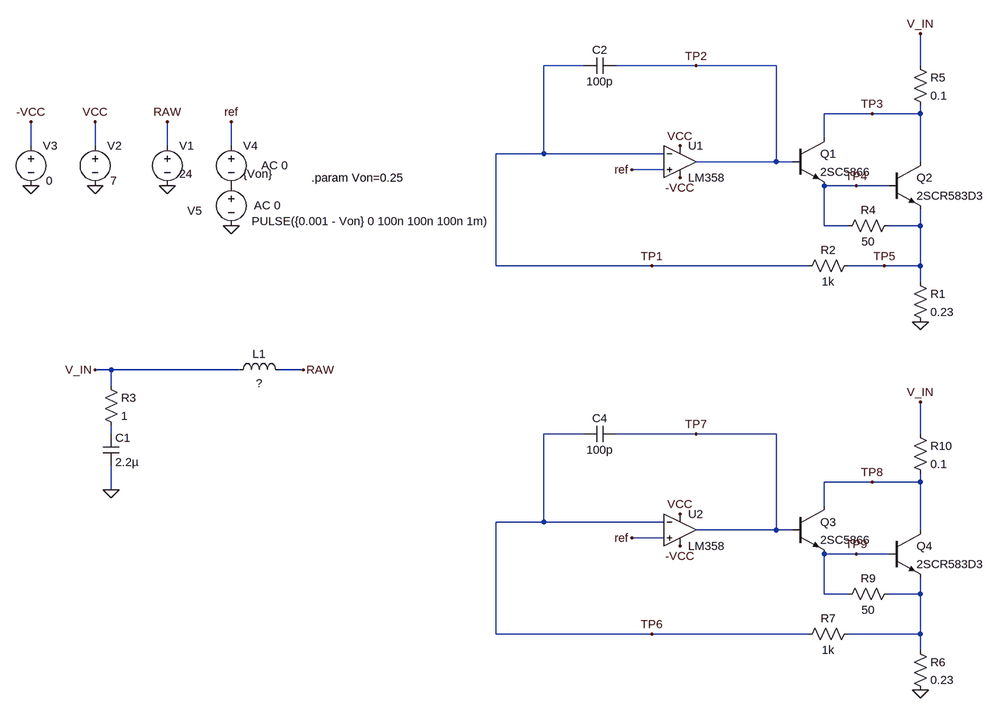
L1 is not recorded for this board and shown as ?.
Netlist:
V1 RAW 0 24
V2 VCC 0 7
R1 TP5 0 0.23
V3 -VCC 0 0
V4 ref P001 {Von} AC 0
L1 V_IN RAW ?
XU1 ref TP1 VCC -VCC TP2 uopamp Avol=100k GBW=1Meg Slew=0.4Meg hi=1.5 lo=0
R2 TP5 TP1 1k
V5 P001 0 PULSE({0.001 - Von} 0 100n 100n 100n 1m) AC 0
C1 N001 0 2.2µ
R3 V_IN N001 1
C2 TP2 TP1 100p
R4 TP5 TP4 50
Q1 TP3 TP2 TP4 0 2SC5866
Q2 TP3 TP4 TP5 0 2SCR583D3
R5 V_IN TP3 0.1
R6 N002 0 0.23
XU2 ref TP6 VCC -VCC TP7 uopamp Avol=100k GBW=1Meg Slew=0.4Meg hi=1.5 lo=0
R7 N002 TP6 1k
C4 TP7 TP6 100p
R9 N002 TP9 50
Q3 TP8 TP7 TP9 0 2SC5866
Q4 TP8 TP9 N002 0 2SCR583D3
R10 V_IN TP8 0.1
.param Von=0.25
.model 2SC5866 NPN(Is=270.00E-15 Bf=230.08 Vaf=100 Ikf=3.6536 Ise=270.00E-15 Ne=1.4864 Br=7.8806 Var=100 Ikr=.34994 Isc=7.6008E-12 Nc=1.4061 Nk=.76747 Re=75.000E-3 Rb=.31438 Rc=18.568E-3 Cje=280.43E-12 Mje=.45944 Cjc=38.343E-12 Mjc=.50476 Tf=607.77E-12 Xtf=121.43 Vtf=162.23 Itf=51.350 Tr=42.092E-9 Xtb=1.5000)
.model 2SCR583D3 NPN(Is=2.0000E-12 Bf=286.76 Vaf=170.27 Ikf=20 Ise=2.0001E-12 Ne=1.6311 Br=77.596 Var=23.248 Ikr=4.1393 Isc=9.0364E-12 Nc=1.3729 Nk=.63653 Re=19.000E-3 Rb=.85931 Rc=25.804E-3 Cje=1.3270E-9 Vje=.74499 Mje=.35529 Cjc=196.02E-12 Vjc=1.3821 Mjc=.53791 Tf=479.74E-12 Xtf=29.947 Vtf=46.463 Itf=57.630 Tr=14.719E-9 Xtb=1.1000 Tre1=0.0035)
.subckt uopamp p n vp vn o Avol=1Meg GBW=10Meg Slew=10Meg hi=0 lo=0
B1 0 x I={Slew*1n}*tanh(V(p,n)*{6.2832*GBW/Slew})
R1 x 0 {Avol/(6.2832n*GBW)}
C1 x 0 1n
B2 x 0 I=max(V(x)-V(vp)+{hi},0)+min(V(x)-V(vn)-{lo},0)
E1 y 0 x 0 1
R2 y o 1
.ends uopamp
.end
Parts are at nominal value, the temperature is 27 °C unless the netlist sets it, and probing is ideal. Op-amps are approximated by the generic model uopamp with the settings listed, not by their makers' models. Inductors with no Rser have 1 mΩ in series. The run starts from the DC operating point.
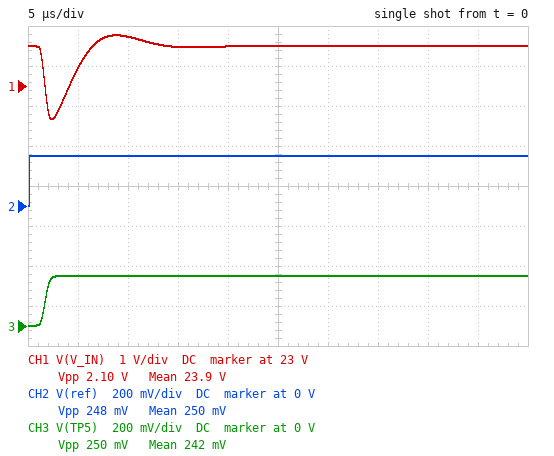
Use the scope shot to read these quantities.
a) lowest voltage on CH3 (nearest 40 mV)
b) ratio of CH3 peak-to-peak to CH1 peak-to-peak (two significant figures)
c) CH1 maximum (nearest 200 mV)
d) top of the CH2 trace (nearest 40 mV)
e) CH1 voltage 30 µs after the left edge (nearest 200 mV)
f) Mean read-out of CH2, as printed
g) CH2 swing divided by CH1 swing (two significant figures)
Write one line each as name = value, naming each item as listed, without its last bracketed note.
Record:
lowest voltage on CH3 = 0 V
ratio of CH3 peak-to-peak to CH1 peak-to-peak = 0.12
CH1 maximum = 24.2 V
top of the CH2 trace = 240 mV
CH1 voltage 30 µs after the left edge = 24.0 V
Mean read-out of CH2, as printed = 250 mV
CH2 swing divided by CH1 swing = 0.12
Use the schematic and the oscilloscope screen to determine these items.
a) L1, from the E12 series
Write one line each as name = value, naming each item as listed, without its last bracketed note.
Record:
L1, from the E12 series = 1.8 µH
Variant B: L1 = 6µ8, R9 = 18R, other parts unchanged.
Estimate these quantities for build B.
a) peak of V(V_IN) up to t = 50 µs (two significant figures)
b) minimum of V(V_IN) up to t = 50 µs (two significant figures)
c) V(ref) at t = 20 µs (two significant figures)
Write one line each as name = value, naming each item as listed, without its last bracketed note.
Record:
peak of V(V_IN) up to t = 50 µs = 25 V
minimum of V(V_IN) up to t = 50 µs = 21 V
V(ref) at t = 20 µs = 250 mV
